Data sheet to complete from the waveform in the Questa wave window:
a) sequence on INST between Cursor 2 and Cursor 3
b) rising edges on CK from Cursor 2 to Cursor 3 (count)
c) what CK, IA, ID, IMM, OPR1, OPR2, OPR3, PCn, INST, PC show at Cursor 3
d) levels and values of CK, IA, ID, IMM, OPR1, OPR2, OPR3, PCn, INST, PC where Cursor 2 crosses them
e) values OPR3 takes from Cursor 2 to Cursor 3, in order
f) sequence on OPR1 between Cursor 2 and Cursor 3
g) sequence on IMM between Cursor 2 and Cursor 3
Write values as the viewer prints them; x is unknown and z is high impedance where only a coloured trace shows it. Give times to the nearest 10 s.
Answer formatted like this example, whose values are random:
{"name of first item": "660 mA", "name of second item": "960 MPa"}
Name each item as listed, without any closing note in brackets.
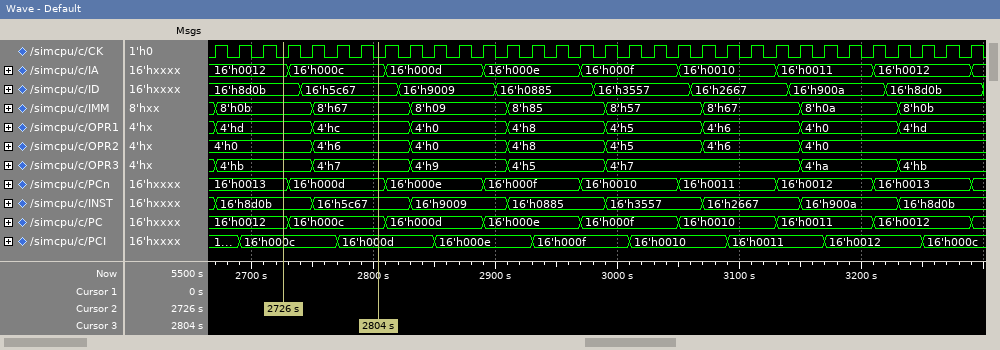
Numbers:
{"sequence on INST between Cursor 2 and Cursor 3": "16'h8d0b, 16'h5c67", "rising edges on CK from Cursor 2 to Cursor 3": "4", "what CK, IA, ID, IMM, OPR1, OPR2, OPR3, PCn, INST, PC show at Cursor 3": "CK=0, IA=16'h000c, ID=16'h5c67, IMM=8'h67, OPR1=4'hc, OPR2=4'h6, OPR3=4'h7, PCn=16'h000d, INST=16'h5c67, PC=16'h000c", "levels and values of CK, IA, ID, IMM, OPR1, OPR2, OPR3, PCn, INST, PC where Cursor 2 crosses them": "CK=0, IA=16'h0012, ID=16'h8d0b, IMM=8'h0b, OPR1=4'hd, OPR2=4'h0, OPR3=4'hb, PCn=16'h0013, INST=16'h8d0b, PC=16'h0012", "values OPR3 takes from Cursor 2 to Cursor 3, in order": "4'hb, 4'h7", "sequence on OPR1 between Cursor 2 and Cursor 3": "4'hd, 4'hc", "sequence on IMM between Cursor 2 and Cursor 3": "8'h0b, 8'h67"}
